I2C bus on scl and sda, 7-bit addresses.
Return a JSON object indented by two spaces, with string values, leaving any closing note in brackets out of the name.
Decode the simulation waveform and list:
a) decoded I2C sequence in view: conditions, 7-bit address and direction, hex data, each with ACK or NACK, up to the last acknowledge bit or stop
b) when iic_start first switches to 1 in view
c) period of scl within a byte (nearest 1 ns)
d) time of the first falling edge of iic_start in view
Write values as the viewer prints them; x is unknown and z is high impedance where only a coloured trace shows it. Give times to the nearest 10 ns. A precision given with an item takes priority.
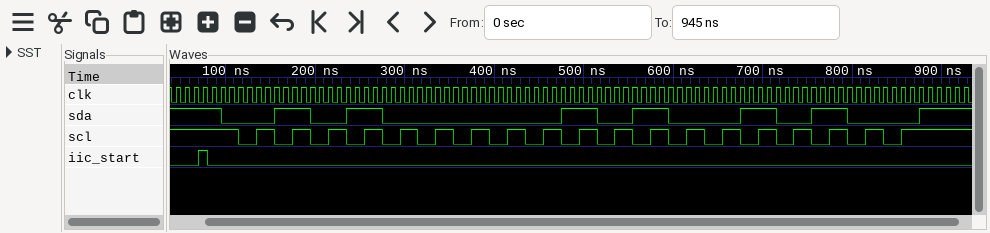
{
  "decoded I2C sequence in view: conditions, 7-bit address and direction, hex data, each with ACK or NACK, up to the last acknowledge bit or stop": "start, address 28 write ACK, A5 ACK, stop",
  "when iic_start first switches to 1 in view": "70 ns",
  "period of scl within a byte": "40 ns",
  "time of the first falling edge of iic_start in view": "80 ns"
}
